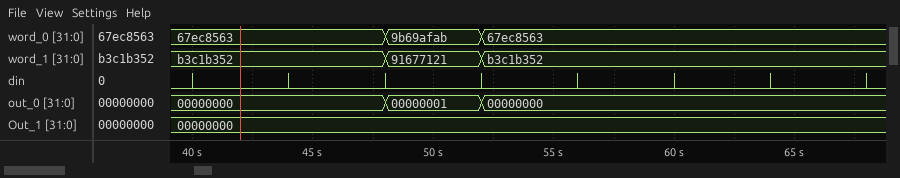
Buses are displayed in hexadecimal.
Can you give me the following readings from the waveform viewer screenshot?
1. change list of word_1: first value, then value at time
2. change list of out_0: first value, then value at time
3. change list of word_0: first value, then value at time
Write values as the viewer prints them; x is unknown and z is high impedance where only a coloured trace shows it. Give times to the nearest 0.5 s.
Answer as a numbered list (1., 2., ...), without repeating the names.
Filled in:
1. b3c1b352, 91677121 at 48 s, b3c1b352 at 52 s
2. 00000000, 00000001 at 48 s, 00000000 at 52 s
3. 67ec8563, 9b69afab at 48 s, 67ec8563 at 52 s
